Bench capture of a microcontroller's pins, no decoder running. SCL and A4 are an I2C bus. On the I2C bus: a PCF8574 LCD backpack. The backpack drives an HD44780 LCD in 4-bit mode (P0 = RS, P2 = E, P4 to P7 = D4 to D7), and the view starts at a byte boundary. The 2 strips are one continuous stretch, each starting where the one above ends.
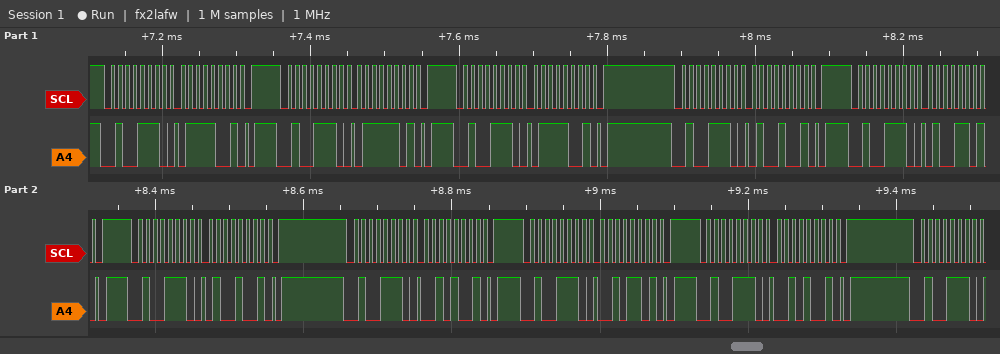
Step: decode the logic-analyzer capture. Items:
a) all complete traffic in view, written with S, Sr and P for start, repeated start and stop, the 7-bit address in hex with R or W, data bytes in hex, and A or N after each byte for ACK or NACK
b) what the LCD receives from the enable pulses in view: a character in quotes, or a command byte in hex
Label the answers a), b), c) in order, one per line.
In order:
a) S 27W A 79 A P S 27W A 7D A P S 27W A 79 A P S 27W A 49 A P S 27W A 4D A P S 27W A 49 A P S 27W A 29 A P S 27W A 2D A P S 27W A 29 A P S 27W A
b) 't'
